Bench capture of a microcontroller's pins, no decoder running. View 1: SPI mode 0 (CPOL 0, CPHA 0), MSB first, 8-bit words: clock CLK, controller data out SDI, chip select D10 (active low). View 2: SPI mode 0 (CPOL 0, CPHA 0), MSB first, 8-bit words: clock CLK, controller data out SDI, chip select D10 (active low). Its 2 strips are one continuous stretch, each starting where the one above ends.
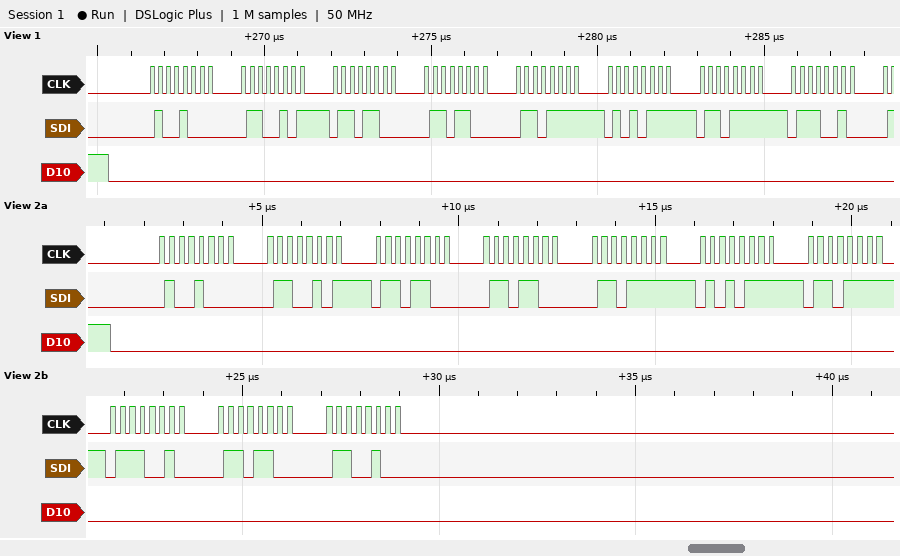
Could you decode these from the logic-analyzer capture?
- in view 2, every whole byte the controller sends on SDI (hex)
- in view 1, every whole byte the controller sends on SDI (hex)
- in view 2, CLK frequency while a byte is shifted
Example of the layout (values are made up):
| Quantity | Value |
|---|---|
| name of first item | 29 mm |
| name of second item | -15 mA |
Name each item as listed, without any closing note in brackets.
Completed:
| Quantity | Value |
|---|---|
| in view 2, every whole byte the controller sends on SDI | 0x48 0x65 0x6C 0x6C 0x6F 0x57 0x6F 0x72 0x6C 0x64 |
| in view 1, every whole byte the controller sends on SDI | 48 65 6C 6C 6F 57 6F 72 |
| in view 2, CLK frequency while a byte is shifted | 4 MHz |
